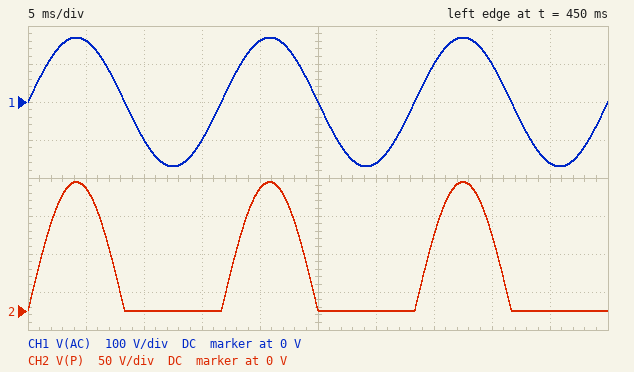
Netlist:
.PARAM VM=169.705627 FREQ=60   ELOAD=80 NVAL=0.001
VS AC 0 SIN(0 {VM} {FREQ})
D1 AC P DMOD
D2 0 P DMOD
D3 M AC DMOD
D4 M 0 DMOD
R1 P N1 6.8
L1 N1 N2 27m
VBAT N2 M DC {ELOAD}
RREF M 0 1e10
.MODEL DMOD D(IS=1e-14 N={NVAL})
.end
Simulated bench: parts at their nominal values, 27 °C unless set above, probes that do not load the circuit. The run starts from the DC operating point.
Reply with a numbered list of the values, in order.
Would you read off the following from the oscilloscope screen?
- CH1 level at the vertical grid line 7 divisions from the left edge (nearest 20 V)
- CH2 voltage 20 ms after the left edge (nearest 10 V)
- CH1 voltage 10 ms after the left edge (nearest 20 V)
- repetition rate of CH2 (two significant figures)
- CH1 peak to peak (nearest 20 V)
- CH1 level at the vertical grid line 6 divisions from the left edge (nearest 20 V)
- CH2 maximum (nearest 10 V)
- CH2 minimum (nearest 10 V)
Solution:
1. 100 V
2. 160 V
3. -100 V
4. 60 Hz
5. 340 V
6. -160 V
7. 170 V
8. 0 V
